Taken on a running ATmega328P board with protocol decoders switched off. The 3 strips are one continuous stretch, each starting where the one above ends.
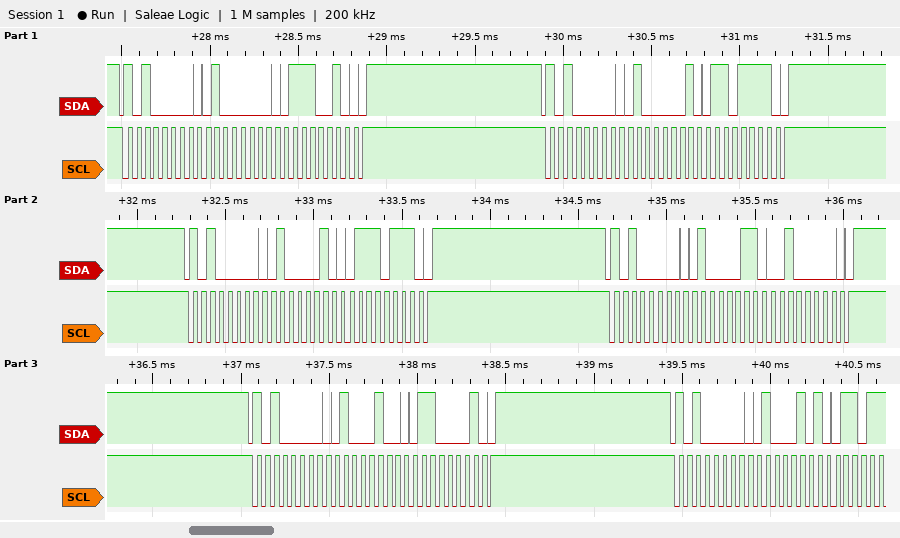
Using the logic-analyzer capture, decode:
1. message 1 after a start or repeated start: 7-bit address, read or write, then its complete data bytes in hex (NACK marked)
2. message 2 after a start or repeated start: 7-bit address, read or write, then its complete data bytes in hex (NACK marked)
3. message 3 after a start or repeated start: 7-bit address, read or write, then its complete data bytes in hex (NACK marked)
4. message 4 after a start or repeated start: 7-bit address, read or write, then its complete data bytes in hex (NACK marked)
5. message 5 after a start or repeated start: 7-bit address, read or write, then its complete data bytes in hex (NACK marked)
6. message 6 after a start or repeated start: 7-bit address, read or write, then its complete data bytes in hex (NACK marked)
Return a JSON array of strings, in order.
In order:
["0x50 write: 40 72", "0x50 write: 41 6F", "0x50 write: 42 77", "0x50 write: 43 20", "0x50 write: 44 61", "0x50 write: 45"]
